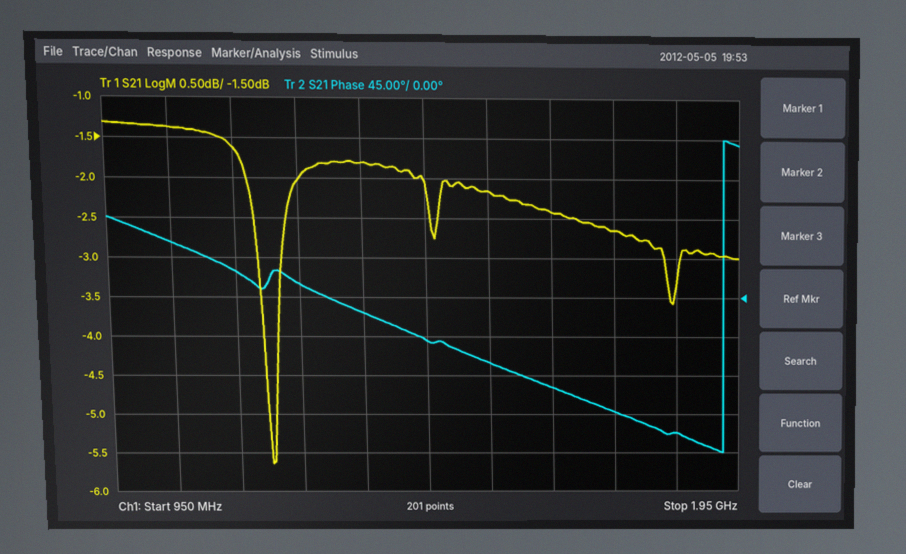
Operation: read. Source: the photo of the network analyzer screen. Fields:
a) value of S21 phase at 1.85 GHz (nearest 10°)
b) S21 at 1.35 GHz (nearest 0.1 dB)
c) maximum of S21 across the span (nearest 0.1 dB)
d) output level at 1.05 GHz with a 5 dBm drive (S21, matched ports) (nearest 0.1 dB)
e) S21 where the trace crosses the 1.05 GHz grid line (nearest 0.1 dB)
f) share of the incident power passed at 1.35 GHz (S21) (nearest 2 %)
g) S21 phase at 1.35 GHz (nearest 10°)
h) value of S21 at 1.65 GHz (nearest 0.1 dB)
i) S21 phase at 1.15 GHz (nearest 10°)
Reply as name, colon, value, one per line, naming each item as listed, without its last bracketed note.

value of S21 phase at 1.85 GHz: -160°
S21 at 1.35 GHz: -1.8 dB
maximum of S21 across the span: -1.3 dB
output level at 1.05 GHz with a 5 dBm drive (S21, matched ports): 3.6 dBm
S21 where the trace crosses the 1.05 GHz grid line: -1.4 dB
share of the incident power passed at 1.35 GHz (S21): 66 %
S21 phase at 1.35 GHz: -20°
value of S21 at 1.65 GHz: -2.4 dB
S21 phase at 1.15 GHz: 30°
